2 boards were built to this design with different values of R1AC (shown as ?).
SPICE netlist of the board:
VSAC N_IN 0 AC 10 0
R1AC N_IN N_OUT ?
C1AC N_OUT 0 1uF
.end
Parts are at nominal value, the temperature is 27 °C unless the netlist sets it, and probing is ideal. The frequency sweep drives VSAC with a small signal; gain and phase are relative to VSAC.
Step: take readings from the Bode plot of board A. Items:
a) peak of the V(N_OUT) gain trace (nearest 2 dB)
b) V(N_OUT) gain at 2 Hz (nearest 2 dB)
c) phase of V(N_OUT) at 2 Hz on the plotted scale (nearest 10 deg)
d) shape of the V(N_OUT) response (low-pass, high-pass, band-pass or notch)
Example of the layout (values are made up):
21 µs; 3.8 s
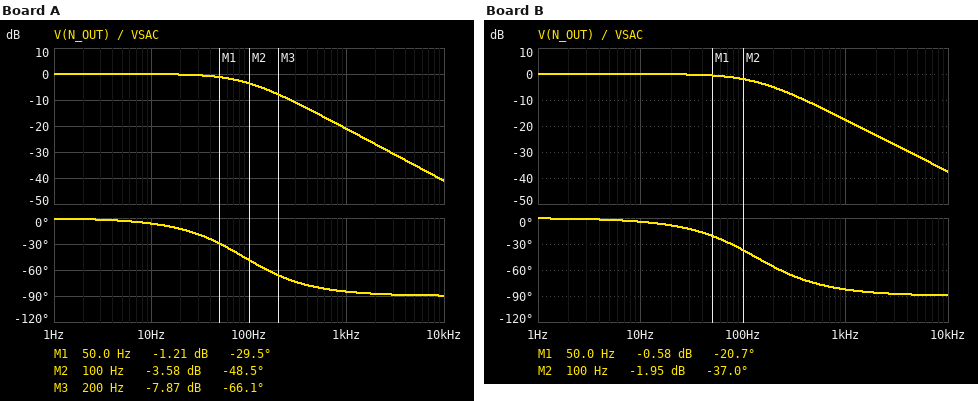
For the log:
0 dB; 0 dB; 0 deg; low-pass
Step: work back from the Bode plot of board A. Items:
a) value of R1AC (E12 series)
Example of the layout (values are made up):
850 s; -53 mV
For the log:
1.8 kΩ
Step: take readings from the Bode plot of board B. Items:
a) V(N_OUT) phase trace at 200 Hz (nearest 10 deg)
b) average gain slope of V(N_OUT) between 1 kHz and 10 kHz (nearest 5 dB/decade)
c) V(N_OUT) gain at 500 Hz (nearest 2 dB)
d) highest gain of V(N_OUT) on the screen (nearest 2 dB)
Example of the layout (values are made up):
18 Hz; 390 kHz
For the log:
-60 deg; -20 dB/decade; -12 dB; 0 dB
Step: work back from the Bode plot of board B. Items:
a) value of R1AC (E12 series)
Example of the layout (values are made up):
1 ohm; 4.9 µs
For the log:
1.2 kΩ
